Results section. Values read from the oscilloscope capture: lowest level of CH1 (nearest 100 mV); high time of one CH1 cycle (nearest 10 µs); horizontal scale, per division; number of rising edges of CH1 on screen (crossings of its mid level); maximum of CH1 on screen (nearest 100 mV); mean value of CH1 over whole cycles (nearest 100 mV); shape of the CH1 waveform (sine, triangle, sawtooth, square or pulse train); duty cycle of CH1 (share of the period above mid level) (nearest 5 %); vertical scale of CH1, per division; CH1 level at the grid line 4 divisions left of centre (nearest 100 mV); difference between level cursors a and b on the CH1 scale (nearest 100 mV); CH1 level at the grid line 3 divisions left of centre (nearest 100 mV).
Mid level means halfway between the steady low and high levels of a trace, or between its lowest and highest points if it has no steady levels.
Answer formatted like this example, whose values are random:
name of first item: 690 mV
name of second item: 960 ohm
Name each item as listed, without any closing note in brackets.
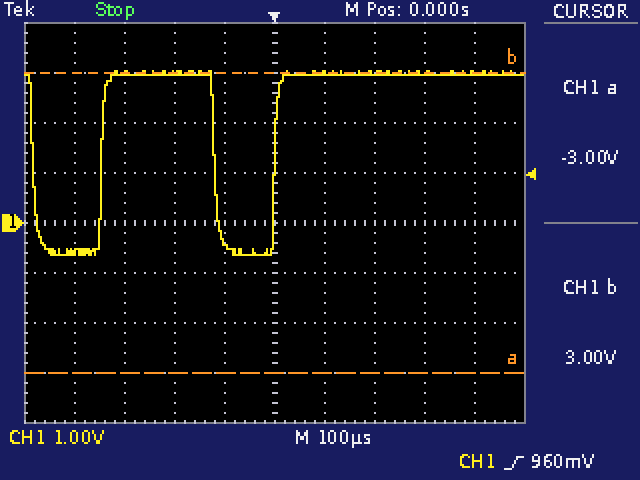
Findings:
lowest level of CH1: -600 mV
high time of one CH1 cycle: 230 µs
horizontal scale, per division: 100 µs
number of rising edges of CH1 on screen: 2
maximum of CH1 on screen: 3.0 V
mean value of CH1 over whole cycles: 1.7 V
shape of the CH1 waveform: pulse train
duty cycle of CH1 (share of the period above mid level): 65 %
vertical scale of CH1, per division: 1 V
CH1 level at the grid line 4 divisions left of centre: -600 mV
difference between level cursors a and b on the CH1 scale: 6.0 V
CH1 level at the grid line 3 divisions left of centre: 3.0 V
